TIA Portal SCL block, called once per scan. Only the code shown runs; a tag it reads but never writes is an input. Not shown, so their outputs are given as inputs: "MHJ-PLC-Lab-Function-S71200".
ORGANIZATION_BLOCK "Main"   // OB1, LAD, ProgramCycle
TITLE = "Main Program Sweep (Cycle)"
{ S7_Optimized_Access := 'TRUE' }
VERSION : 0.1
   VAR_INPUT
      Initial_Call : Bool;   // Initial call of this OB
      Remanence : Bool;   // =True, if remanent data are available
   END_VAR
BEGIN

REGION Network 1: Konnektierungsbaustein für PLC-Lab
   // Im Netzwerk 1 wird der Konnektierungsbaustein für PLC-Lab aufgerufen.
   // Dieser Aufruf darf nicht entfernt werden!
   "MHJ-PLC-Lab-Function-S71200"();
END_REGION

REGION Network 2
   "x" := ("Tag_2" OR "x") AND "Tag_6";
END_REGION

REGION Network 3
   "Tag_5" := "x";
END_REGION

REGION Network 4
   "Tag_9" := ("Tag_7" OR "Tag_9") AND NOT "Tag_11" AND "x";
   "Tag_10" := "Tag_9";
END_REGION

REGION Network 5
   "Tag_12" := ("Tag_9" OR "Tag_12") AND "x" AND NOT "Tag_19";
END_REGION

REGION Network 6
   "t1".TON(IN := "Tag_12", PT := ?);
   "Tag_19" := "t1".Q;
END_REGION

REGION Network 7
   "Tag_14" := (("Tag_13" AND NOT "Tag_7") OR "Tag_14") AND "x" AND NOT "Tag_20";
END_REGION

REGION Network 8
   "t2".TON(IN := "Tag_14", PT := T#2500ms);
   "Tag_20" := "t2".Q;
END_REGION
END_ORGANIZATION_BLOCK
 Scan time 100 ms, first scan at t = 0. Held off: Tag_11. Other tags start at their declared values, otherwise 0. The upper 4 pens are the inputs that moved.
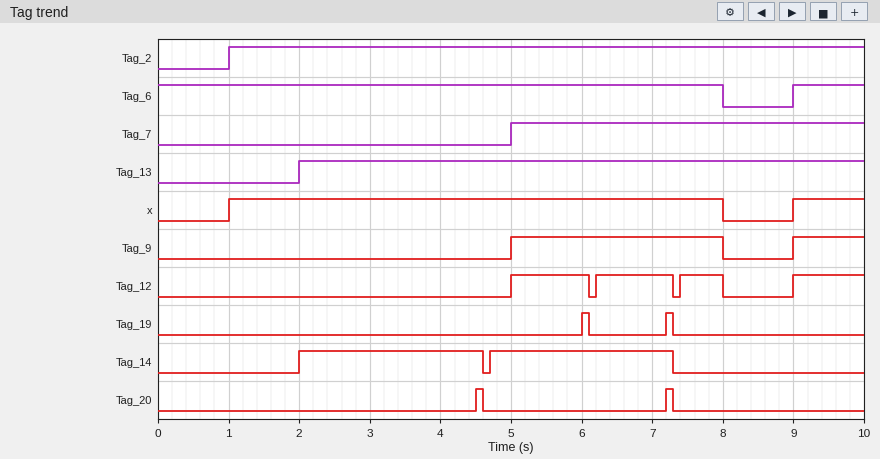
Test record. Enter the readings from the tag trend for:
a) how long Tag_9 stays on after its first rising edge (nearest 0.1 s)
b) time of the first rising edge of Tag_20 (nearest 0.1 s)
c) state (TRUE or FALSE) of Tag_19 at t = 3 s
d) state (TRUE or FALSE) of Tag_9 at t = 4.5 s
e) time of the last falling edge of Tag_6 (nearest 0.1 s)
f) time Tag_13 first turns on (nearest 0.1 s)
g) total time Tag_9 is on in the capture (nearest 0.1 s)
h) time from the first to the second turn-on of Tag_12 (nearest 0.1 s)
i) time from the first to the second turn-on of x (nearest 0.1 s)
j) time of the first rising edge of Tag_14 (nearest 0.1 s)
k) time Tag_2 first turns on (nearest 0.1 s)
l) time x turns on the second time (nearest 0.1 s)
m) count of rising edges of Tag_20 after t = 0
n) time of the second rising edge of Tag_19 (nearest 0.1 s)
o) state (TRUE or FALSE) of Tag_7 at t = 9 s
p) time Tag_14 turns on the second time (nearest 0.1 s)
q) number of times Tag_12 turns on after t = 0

3.0 s
4.5 s
FALSE
FALSE
8.0 s
2.0 s
4.0 s
1.2 s
8.0 s
2.0 s
1.0 s
9.0 s
2
7.2 s
TRUE
4.7 s
4
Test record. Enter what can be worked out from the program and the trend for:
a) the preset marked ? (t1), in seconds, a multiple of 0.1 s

1.0 s
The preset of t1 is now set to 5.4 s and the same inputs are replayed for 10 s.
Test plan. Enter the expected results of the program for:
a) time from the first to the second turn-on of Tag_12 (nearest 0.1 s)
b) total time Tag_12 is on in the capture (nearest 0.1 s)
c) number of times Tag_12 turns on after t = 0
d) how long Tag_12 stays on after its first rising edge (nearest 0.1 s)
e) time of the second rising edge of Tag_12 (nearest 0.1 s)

4.0 s
4.0 s
2
3.0 s
9.0 s
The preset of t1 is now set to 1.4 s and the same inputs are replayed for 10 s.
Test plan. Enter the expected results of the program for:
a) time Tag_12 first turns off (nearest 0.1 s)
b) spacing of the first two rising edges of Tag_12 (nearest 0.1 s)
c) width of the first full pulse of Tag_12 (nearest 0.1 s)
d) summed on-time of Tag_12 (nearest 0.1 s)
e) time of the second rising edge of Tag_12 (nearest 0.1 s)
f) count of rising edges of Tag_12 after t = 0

6.5 s
1.6 s
1.5 s
3.9 s
6.6 s
3
